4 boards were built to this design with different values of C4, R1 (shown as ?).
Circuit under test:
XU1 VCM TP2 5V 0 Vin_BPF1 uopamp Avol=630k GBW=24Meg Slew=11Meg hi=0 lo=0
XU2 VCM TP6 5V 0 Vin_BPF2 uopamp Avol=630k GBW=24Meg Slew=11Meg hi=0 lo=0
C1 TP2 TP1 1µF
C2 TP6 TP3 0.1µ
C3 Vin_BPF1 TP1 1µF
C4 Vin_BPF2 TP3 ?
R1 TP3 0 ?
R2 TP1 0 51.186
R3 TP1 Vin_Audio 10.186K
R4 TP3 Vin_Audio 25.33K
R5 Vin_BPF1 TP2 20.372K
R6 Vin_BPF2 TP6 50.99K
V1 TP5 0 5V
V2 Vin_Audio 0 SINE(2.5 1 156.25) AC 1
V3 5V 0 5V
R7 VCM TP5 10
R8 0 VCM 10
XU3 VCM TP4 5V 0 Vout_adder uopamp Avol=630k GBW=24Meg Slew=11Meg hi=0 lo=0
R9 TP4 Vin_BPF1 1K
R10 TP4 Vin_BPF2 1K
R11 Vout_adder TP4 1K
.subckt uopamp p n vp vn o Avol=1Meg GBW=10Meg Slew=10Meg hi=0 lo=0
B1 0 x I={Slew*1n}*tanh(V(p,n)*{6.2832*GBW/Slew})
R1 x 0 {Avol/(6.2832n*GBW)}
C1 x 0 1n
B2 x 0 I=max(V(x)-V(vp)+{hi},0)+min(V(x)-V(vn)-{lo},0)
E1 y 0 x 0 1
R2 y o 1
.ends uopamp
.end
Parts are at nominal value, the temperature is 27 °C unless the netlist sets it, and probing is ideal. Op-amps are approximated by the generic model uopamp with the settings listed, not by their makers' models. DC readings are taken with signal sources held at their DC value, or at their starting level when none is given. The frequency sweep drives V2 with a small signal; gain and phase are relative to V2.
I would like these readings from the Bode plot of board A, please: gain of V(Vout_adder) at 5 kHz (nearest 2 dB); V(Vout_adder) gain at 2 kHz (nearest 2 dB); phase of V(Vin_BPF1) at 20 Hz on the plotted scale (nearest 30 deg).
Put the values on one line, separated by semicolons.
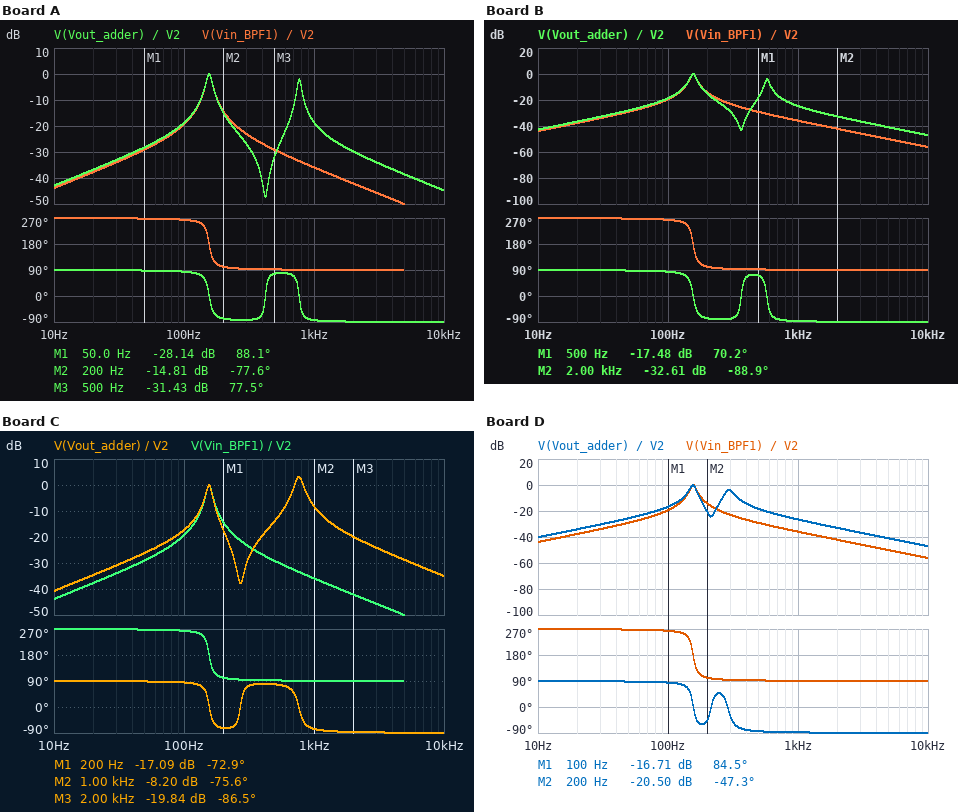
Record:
-38 dB; -30 dB; 270 deg
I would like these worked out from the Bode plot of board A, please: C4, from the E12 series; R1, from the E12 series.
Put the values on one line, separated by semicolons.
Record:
150 nF; 56 Ω
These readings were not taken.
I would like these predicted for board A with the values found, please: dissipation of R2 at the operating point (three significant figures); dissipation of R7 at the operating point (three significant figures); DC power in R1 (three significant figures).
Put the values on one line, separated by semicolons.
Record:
3.05 µW; 625 mW; 543 nW
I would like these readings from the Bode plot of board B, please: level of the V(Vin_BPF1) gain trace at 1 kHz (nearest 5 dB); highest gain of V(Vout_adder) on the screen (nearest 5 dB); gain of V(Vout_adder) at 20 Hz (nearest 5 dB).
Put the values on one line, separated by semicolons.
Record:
-35 dB; 0 dB; -35 dB
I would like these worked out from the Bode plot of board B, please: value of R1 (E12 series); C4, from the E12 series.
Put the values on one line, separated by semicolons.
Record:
68 Ω; 220 nF
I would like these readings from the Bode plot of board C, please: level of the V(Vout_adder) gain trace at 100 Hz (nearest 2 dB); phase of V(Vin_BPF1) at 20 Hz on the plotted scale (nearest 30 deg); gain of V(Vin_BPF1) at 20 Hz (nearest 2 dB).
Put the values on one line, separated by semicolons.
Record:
-18 dB; 270 deg; -38 dB
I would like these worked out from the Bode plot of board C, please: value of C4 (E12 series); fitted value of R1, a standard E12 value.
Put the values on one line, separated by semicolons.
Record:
39 nF; 220 Ω
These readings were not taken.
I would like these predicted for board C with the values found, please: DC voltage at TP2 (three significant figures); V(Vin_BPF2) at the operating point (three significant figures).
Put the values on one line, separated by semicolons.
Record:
2.50 V; 2.50 V
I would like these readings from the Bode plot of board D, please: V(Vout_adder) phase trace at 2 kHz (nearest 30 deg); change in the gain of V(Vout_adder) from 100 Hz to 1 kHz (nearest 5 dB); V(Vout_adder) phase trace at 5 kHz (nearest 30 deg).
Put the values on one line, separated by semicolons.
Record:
-90 deg; -10 dB; -90 deg
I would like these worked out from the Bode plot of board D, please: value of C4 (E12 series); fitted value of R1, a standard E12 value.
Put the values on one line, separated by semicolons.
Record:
220 nF; 270 Ω
